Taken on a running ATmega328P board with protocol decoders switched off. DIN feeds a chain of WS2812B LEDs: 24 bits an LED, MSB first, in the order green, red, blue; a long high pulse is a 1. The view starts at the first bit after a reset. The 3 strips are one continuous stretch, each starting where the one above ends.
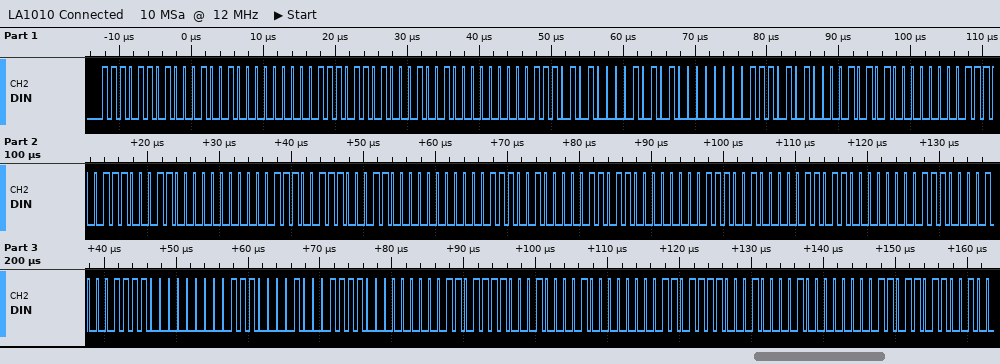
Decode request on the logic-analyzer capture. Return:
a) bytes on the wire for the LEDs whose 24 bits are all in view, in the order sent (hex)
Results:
ED 12 00 ED 12 00 EA 15 00 EA 15 00 E7 18 00 E7 18 00 E4 1B 00 E4 1B 00 E1 1E 00 E1 1E 00 DE 21 00 DE 21 00
